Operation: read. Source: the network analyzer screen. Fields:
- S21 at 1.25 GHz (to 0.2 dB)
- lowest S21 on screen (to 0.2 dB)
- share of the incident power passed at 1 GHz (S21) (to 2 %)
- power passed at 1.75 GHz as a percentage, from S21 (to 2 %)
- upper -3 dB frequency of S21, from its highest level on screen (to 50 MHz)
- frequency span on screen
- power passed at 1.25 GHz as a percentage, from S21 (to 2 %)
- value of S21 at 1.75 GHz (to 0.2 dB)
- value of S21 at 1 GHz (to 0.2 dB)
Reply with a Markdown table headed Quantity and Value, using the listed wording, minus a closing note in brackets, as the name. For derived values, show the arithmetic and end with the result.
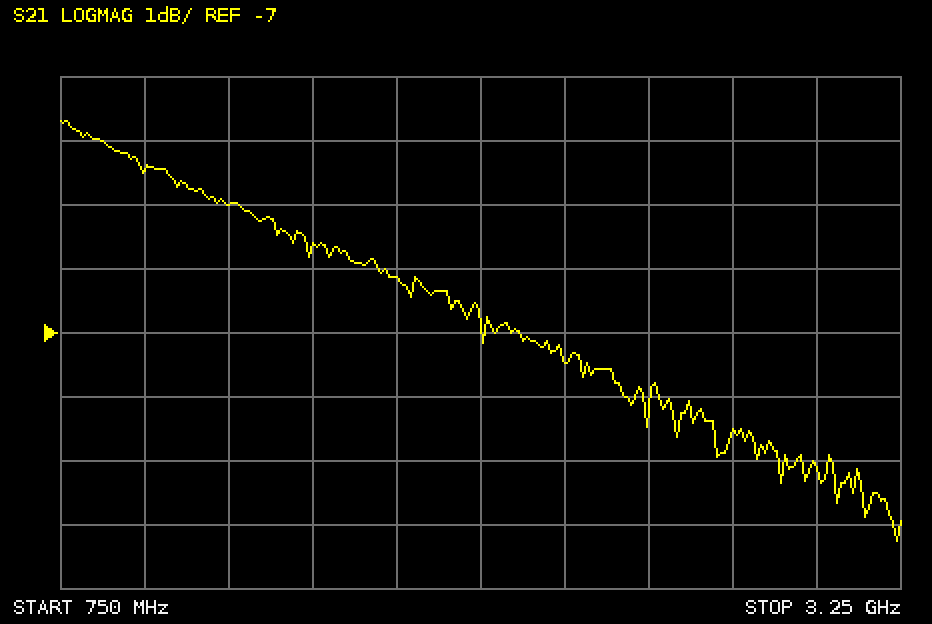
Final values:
| Quantity | Value |
|---|---|
| S21 at 1.25 GHz | -5.0 dB |
| lowest S21 on screen | -10.2 dB |
| share of the incident power passed at 1 GHz (S21) | 10^(-4.4/10) ≈ 36 % |
| power passed at 1.75 GHz as a percentage, from S21 | 10^(-6.2/10) ≈ 24 % |
| upper -3 dB frequency of S21, from its highest level on screen | 1.95 GHz |
| frequency span on screen | 2.5 GHz |
| power passed at 1.25 GHz as a percentage, from S21 | 10^(-5/10) ≈ 32 % |
| value of S21 at 1.75 GHz | -6.2 dB |
| value of S21 at 1 GHz | -4.4 dB |
